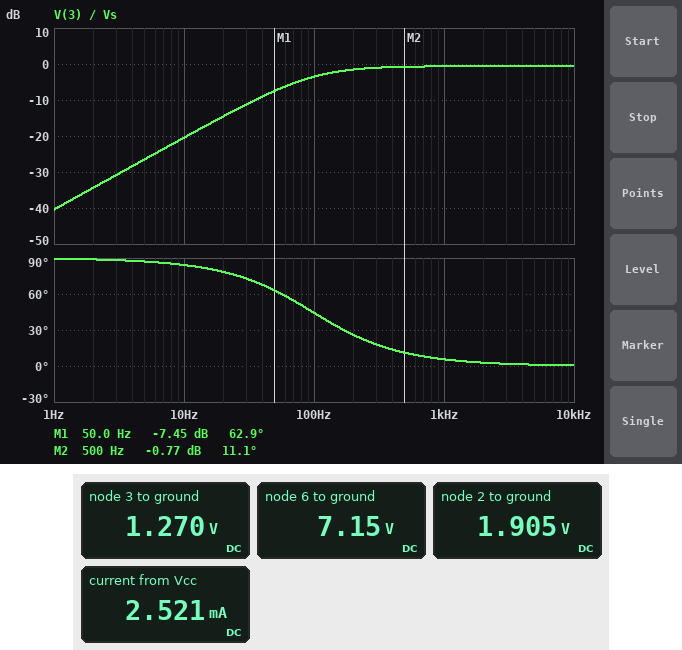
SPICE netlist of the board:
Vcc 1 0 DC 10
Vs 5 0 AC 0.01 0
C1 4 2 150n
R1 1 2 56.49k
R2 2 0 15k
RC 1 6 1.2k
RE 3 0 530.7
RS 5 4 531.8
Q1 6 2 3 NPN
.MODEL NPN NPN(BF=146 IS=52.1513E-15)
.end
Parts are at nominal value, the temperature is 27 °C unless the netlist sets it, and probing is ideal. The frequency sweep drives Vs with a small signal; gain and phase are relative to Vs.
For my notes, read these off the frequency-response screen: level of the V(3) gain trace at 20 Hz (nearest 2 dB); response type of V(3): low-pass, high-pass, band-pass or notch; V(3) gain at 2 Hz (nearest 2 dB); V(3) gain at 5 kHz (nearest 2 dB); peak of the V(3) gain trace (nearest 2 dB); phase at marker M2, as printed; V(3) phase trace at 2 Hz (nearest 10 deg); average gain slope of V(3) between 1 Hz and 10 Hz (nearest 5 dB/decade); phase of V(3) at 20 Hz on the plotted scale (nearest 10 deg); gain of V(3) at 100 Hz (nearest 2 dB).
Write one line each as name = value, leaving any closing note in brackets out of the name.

level of the V(3) gain trace at 20 Hz = -14 dB
response type of V(3): low-pass, high-pass, band-pass or notch = high-pass
V(3) gain at 2 Hz = -34 dB
V(3) gain at 5 kHz = 0 dB
peak of the V(3) gain trace = 0 dB
phase at marker M2, as printed = 11.1 deg
V(3) phase trace at 2 Hz = 90 deg
average gain slope of V(3) between 1 Hz and 10 Hz = 20 dB/decade
phase of V(3) at 20 Hz on the plotted scale = 80 deg
gain of V(3) at 100 Hz = -4 dB
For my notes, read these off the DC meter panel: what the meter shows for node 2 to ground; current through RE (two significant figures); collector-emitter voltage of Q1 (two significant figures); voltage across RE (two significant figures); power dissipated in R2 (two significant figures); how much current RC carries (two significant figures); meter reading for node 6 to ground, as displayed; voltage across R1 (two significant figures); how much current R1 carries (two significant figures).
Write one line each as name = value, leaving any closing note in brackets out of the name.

what the meter shows for node 2 to ground = 1.905 V
current through RE = 2.4 mA
collector-emitter voltage of Q1 = 5.9 V
voltage across RE = 1.3 V
power dissipated in R2 = 240 µW
how much current RC carries = 2.4 mA
meter reading for node 6 to ground, as displayed = 7.15 V
voltage across R1 = 8.1 V
how much current R1 carries = 140 µA
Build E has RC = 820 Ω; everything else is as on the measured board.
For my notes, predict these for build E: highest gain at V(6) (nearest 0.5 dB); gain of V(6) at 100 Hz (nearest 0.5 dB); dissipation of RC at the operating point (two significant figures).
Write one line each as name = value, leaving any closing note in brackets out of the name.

highest gain at V(6) = 3.0 dB
gain of V(6) at 100 Hz = 0 dB
dissipation of RC at the operating point = 4.6 mW
